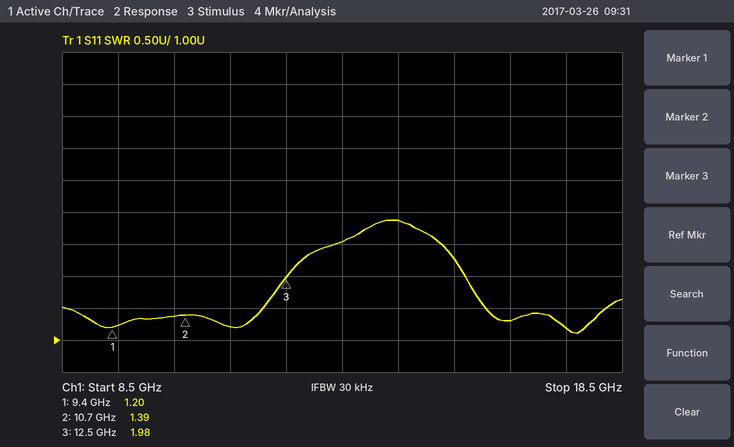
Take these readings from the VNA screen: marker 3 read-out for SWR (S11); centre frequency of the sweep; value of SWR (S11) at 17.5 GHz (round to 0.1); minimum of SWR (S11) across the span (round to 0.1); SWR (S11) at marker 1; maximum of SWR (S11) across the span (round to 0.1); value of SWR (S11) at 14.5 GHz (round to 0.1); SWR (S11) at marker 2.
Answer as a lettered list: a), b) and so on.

a) 1.98
b) 13.5 GHz
c) 1.2
d) 1.1
e) 1.20
f) 2.9
g) 2.9
h) 1.39
